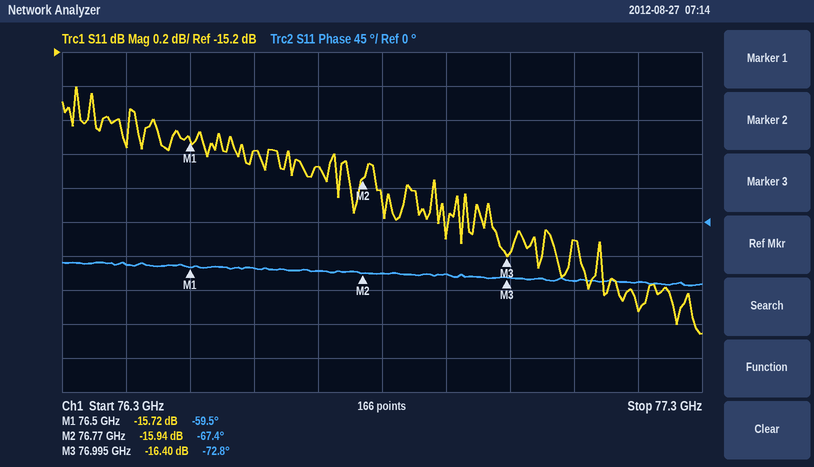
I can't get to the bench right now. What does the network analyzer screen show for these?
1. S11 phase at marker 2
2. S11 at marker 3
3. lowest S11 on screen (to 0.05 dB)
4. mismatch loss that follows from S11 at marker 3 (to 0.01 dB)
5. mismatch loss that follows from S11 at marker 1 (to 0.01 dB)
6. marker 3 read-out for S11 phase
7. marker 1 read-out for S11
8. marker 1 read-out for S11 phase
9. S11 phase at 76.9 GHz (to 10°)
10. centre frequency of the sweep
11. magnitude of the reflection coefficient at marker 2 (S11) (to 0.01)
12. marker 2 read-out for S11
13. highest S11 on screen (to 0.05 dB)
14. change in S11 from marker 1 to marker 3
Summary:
-67.4°
-16.40 dB
-16.85 dB
0.10 dB
0.12 dB
-72.8°
-15.72 dB
-59.5°
-70°
76.8 GHz
0.16
-15.94 dB
-15.40 dB
-0.68 dB
